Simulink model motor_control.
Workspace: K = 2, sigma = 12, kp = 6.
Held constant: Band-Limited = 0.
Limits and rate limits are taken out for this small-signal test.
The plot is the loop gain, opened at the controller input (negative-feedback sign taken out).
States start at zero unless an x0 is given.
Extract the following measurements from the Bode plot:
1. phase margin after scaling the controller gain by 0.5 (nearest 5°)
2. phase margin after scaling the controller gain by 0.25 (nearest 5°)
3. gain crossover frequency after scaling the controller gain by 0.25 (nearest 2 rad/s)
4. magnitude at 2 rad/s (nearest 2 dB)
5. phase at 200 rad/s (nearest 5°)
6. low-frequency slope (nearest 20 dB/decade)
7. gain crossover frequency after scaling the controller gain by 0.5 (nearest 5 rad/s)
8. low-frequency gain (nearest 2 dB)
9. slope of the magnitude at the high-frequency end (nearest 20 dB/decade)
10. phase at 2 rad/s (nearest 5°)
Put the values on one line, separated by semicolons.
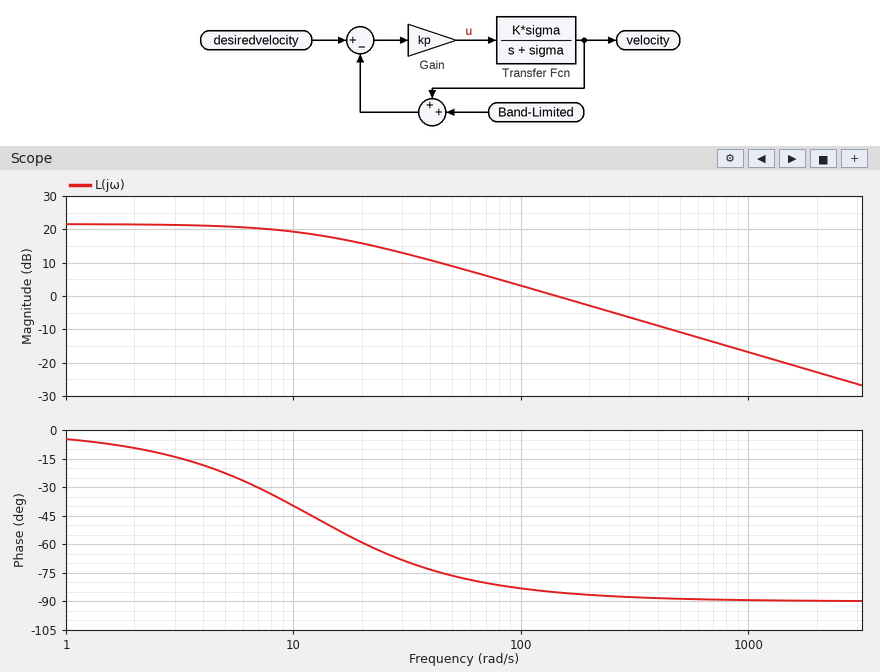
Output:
100°; 110°; 34 rad/s; 22 dB; -85°; 0 dB/decade; 70 rad/s; 22 dB; -20 dB/decade; -10°
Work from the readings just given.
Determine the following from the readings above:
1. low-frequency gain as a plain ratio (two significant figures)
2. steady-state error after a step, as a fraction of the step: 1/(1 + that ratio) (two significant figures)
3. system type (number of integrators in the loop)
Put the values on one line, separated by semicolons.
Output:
13; 0.071; 0
